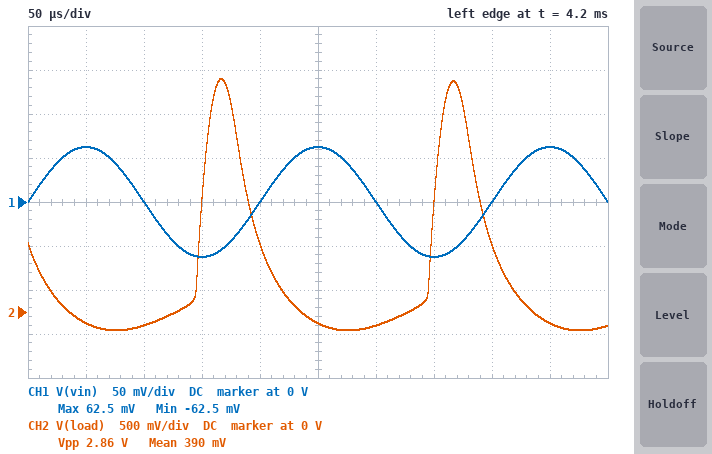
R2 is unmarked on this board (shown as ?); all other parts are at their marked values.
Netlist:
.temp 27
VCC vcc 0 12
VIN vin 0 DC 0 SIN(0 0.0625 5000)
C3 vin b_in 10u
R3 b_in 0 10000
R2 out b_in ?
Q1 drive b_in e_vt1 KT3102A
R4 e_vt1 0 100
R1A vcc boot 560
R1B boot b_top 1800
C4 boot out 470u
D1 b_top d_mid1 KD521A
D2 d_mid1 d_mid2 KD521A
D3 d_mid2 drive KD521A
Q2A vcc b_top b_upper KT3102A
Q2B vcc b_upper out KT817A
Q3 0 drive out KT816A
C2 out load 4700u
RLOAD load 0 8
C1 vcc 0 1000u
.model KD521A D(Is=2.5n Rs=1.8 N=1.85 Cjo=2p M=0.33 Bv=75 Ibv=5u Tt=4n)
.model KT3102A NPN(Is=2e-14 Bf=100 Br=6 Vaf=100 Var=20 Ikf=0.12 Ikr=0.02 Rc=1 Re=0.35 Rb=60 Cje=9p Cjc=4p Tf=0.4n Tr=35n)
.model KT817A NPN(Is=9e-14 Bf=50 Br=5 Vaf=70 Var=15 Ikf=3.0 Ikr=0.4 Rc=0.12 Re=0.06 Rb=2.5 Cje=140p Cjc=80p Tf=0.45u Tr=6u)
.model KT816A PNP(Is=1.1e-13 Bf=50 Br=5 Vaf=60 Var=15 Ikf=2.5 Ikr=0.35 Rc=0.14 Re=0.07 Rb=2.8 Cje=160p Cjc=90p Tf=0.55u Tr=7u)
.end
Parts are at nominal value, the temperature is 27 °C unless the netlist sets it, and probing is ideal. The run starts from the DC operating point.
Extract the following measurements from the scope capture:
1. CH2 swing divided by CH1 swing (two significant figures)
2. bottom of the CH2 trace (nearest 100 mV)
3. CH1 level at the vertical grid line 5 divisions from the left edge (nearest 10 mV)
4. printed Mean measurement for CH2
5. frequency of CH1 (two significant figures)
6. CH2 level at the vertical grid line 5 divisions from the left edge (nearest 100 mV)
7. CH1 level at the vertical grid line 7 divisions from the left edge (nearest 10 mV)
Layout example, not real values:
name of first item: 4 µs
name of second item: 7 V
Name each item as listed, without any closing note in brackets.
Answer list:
CH2 swing divided by CH1 swing: 23
bottom of the CH2 trace: -200 mV
CH1 level at the vertical grid line 5 divisions from the left edge: 60 mV
printed Mean measurement for CH2: 390 mV
frequency of CH1: 5.0 kHz
CH2 level at the vertical grid line 5 divisions from the left edge: -100 mV
CH1 level at the vertical grid line 7 divisions from the left edge: -60 mV
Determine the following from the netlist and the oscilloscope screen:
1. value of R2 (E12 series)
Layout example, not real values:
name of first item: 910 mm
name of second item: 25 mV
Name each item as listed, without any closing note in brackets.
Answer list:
value of R2: 68 kΩ
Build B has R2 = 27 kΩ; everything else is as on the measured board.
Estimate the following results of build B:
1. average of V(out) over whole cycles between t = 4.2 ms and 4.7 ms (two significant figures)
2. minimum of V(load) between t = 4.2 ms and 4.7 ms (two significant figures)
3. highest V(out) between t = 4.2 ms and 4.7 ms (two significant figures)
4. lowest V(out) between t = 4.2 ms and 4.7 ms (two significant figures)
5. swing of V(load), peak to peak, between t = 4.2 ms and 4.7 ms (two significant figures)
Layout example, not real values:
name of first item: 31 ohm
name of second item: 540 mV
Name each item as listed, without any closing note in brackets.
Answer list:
average of V(out) over whole cycles between t = 4.2 ms and 4.7 ms: 4.6 V
minimum of V(load) between t = 4.2 ms and 4.7 ms: -230 mV
highest V(out) between t = 4.2 ms and 4.7 ms: 4.9 V
lowest V(out) between t = 4.2 ms and 4.7 ms: 4.4 V
swing of V(load), peak to peak, between t = 4.2 ms and 4.7 ms: 530 mV
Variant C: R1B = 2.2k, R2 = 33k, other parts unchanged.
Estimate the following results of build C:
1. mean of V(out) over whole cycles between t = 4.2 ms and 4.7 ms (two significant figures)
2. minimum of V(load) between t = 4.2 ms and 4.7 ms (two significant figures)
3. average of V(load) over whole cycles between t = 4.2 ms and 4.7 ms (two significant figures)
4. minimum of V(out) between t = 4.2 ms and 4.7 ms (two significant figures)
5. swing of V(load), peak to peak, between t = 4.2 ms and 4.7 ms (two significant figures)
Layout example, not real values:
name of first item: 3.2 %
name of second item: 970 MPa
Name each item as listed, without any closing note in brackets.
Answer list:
mean of V(out) over whole cycles between t = 4.2 ms and 4.7 ms: 4.9 V
minimum of V(load) between t = 4.2 ms and 4.7 ms: -220 mV
average of V(load) over whole cycles between t = 4.2 ms and 4.7 ms: 44 mV
minimum of V(out) between t = 4.2 ms and 4.7 ms: 4.6 V
swing of V(load), peak to peak, between t = 4.2 ms and 4.7 ms: 630 mV
